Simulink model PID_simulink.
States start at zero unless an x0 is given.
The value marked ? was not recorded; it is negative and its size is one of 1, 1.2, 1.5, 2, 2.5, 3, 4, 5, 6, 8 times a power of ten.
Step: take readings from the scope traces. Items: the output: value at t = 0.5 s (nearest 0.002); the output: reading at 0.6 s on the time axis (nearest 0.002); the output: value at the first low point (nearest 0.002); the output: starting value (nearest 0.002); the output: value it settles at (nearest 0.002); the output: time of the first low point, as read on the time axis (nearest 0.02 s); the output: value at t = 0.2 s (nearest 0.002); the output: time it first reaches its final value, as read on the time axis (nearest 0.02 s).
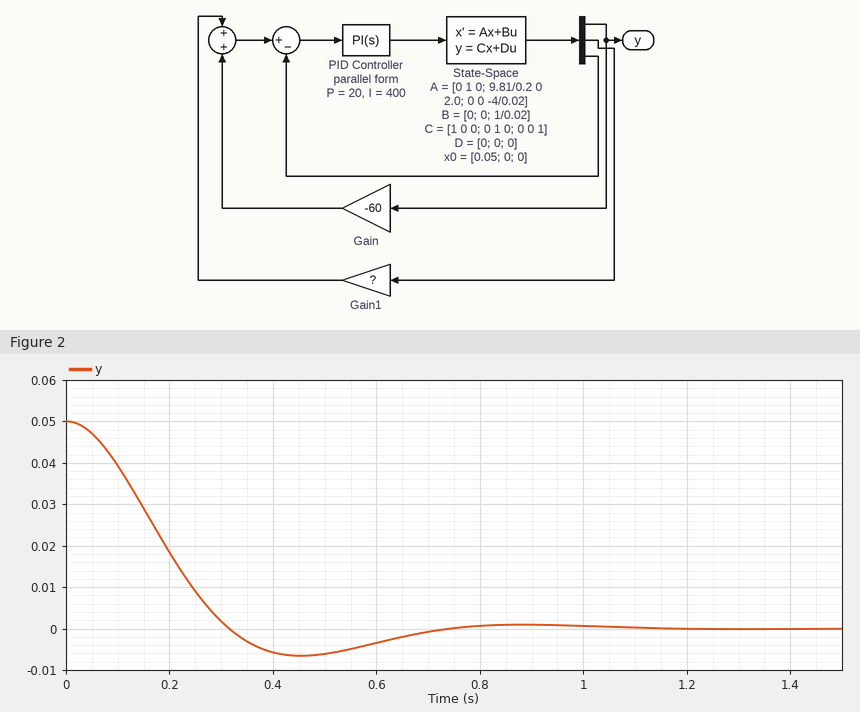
-0.006
-0.004
-0.006
0.050
0.000
0.46 s
0.018
0.32 s
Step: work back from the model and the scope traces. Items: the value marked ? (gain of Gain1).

-5
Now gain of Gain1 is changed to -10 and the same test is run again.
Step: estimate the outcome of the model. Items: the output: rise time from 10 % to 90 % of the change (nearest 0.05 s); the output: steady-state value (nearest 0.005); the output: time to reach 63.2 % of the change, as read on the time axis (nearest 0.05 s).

0.50 s
0.000
0.30 s
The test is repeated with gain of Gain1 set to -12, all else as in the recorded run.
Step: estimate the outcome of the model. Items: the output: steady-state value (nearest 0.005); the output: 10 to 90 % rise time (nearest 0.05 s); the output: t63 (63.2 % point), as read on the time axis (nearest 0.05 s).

0.000
0.65 s
0.35 s
